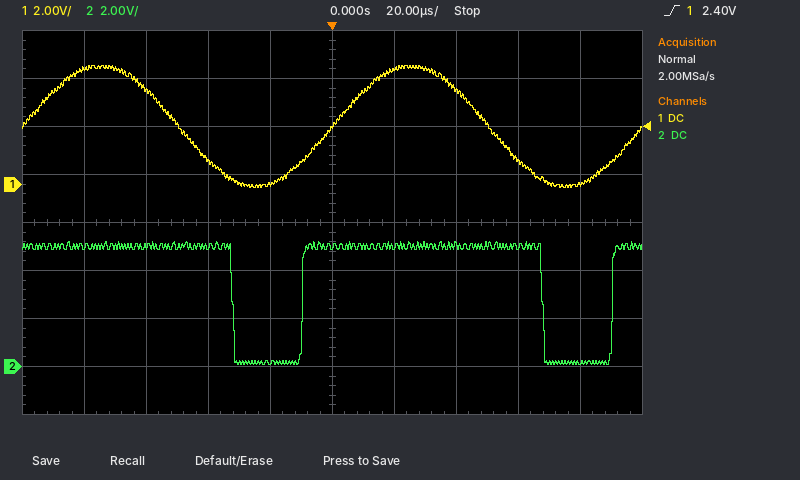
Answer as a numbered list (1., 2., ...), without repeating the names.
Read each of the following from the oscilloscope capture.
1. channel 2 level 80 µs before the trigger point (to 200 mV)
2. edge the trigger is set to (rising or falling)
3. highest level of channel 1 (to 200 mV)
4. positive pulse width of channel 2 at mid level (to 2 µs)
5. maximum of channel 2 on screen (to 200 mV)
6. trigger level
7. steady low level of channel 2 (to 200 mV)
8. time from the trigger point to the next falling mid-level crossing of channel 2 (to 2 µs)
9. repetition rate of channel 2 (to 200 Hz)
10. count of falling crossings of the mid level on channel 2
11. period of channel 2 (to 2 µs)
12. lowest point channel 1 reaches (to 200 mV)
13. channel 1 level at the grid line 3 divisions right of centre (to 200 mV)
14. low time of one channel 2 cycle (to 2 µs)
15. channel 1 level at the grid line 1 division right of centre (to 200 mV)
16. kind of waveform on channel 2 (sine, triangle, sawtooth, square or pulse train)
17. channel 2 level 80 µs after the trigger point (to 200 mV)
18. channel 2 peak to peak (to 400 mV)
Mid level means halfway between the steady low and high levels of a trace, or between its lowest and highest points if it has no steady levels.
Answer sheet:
1. 5.0 V
2. rising
3. 5.0 V
4. 78 µs
5. 5.2 V
6. 2.40 V
7. 200 mV
8. 68 µs
9. 10.0 kHz
10. 2
11. 100 µs
12. -200 mV
13. 1.0 V
14. 22 µs
15. 4.8 V
16. pulse train
17. 200 mV
18. 5.2 V
